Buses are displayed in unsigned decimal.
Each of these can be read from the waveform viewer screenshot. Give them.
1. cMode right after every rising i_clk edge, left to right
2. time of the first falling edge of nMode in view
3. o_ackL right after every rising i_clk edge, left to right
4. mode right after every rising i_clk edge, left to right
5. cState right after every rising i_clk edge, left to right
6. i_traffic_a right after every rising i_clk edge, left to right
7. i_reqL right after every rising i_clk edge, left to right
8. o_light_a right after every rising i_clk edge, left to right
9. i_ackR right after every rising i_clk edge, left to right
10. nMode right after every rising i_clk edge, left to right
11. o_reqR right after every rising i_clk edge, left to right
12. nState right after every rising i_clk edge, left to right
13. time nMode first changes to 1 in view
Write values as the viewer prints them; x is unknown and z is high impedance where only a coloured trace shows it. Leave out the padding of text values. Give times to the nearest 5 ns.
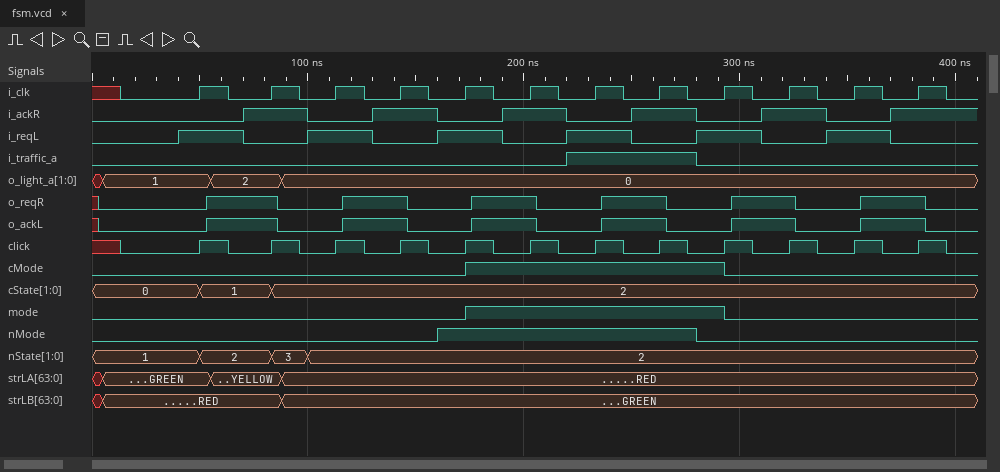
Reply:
0 0 0 0 1 1 1 1 0 0 0 0
280 ns
0 1 0 1 0 1 0 1 0 1 0 1
0 0 0 0 1 1 1 1 0 0 0 0
1, 2, 2, 2, 2, 2, 2, 2, 2, 2, 2, 2
0 0 0 0 0 0 1 1 0 0 0 0
1 0 1 0 1 0 1 0 1 0 1 0
1, 2, 0, 0, 0, 0, 0, 0, 0, 0, 0, 0
0 1 0 1 0 1 0 1 0 1 0 1
0 0 0 0 1 1 1 1 0 0 0 0
0 1 0 1 0 1 0 1 0 1 0 1
2, 3, 2, 2, 2, 2, 2, 2, 2, 2, 2, 2
160 ns
